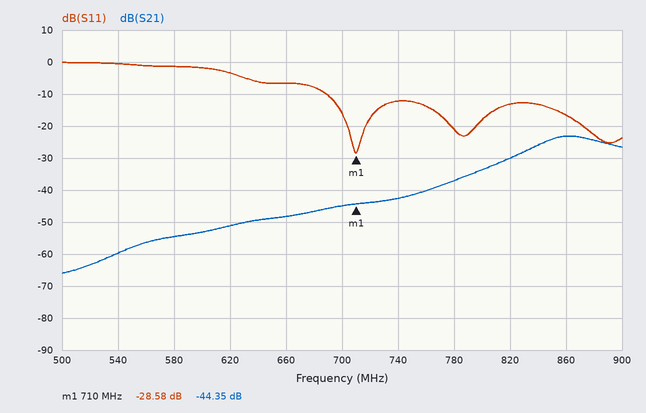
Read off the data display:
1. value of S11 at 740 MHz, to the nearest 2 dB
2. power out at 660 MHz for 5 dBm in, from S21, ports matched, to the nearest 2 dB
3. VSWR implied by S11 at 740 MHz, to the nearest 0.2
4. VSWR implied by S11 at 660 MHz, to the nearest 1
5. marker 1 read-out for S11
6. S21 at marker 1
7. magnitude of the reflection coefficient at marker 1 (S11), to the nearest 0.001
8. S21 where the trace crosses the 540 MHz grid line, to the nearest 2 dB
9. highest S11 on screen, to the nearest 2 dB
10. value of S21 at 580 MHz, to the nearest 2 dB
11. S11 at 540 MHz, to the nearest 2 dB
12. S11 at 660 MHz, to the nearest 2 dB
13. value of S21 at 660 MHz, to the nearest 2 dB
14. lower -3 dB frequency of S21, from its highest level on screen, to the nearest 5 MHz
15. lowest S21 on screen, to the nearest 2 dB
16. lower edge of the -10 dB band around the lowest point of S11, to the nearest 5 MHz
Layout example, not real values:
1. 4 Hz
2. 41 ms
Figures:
1. -12 dB
2. -44 dBm
3. 1.6
4. 3
5. -28.58 dB
6. -44.35 dB
7. 0.037
8. -60 dB
9. 0 dB
10. -54 dB
11. 0 dB
12. -6 dB
13. -48 dB
14. 840 MHz
15. -66 dB
16. 690 MHz
